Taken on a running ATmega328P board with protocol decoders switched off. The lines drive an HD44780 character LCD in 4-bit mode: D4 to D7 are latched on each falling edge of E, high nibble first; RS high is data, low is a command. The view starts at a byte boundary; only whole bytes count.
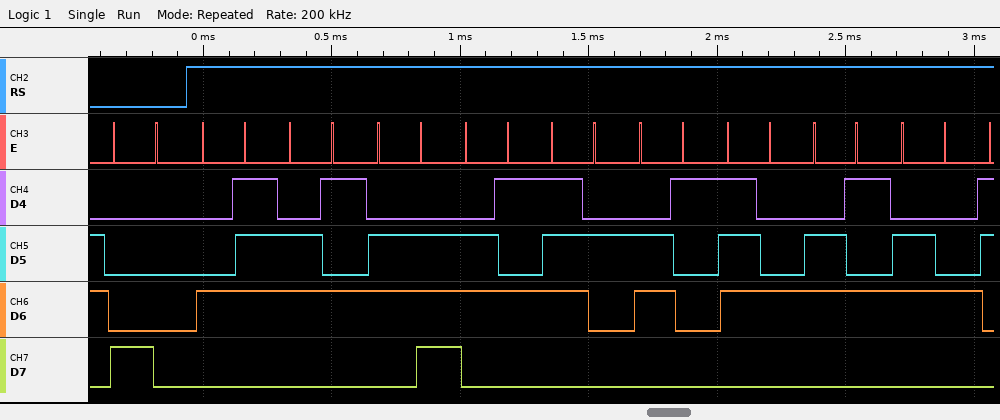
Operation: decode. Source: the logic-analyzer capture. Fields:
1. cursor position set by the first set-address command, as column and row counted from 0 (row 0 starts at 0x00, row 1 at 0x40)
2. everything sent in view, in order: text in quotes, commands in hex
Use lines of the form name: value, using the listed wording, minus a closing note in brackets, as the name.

cursor position set by the first set-address command, as column and row counted from 0: column 0, row 0
everything sent in view, in order: text in quotes, commands in hex: 0x80 "Generated"
